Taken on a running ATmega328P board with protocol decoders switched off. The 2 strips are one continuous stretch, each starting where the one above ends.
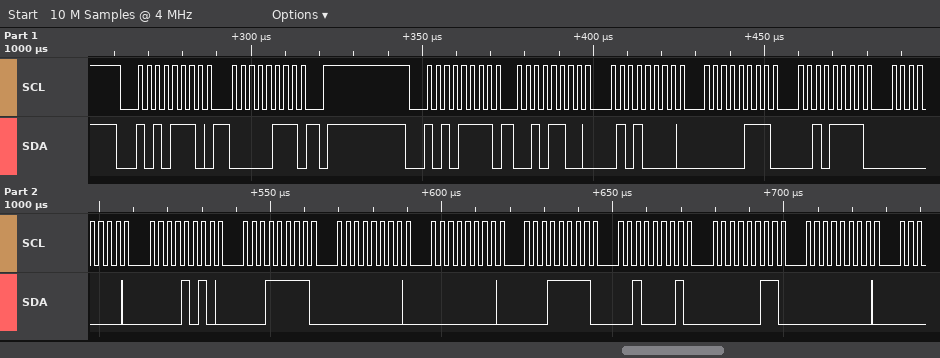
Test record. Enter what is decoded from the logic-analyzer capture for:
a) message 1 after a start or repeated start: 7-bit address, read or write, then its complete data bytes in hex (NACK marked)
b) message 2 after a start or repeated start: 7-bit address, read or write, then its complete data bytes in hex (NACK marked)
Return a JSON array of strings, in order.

["0x57 write: 07", "0x57 read: 2C 50 07 2F 00 0A 1F 00 00 1F 21 03 00"]
